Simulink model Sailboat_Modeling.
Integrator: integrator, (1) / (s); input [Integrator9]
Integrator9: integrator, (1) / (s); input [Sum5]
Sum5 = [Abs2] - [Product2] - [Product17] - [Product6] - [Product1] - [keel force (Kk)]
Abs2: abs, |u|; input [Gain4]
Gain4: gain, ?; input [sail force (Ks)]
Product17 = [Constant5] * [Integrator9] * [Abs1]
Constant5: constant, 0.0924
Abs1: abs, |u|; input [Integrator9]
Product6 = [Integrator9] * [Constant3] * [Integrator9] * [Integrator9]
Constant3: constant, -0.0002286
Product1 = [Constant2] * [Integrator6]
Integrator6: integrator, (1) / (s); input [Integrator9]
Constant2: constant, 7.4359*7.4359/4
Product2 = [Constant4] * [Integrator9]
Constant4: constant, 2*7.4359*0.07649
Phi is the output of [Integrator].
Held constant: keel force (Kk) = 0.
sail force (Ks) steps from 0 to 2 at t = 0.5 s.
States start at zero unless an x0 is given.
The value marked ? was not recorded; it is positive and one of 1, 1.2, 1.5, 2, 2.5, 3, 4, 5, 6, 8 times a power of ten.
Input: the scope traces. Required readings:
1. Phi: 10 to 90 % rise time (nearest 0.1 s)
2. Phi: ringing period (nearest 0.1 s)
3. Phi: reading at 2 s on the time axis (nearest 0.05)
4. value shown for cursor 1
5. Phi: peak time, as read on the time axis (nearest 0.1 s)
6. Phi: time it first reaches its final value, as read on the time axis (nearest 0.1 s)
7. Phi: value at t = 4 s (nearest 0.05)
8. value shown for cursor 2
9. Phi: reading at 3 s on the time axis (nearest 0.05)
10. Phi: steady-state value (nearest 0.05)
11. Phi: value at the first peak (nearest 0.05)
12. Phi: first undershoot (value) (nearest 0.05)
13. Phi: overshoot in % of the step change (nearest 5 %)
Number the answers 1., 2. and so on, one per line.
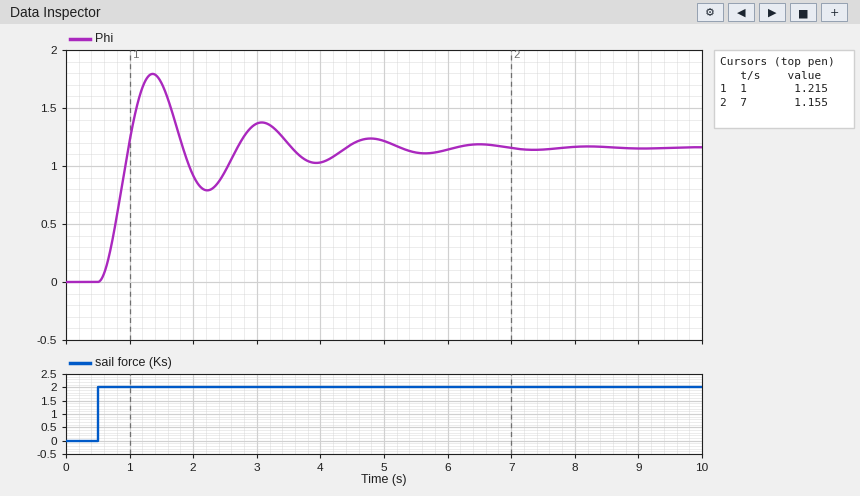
1. 0.3 s
2. 1.7 s
3. 0.90
4. 1.215
5. 1.4 s
6. 1.0 s
7. 1.05
8. 1.155
9. 1.35
10. 1.15
11. 1.80
12. 0.80
13. 55 %
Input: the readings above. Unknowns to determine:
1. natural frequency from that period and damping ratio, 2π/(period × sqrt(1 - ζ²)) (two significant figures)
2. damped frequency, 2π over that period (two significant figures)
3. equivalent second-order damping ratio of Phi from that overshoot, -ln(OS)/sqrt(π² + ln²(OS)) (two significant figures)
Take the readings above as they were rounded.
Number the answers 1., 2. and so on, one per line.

1. 3.8 rad/s
2. 3.7 rad/s
3. 0.19
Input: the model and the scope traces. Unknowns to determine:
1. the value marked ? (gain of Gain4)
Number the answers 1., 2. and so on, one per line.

1. 8
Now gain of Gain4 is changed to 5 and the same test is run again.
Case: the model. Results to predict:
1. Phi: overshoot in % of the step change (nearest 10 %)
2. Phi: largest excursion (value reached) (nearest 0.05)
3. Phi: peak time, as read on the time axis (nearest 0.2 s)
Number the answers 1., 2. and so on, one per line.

1. 60 %
2. 1.15
3. 1.4 s
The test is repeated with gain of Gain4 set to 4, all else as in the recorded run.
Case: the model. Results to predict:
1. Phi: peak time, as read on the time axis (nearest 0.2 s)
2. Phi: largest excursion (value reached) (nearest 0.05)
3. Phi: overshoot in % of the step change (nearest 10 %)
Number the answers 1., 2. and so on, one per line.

1. 1.4 s
2. 0.90
3. 60 %
